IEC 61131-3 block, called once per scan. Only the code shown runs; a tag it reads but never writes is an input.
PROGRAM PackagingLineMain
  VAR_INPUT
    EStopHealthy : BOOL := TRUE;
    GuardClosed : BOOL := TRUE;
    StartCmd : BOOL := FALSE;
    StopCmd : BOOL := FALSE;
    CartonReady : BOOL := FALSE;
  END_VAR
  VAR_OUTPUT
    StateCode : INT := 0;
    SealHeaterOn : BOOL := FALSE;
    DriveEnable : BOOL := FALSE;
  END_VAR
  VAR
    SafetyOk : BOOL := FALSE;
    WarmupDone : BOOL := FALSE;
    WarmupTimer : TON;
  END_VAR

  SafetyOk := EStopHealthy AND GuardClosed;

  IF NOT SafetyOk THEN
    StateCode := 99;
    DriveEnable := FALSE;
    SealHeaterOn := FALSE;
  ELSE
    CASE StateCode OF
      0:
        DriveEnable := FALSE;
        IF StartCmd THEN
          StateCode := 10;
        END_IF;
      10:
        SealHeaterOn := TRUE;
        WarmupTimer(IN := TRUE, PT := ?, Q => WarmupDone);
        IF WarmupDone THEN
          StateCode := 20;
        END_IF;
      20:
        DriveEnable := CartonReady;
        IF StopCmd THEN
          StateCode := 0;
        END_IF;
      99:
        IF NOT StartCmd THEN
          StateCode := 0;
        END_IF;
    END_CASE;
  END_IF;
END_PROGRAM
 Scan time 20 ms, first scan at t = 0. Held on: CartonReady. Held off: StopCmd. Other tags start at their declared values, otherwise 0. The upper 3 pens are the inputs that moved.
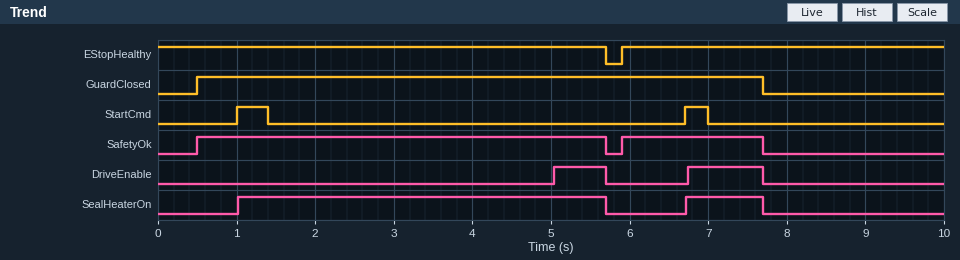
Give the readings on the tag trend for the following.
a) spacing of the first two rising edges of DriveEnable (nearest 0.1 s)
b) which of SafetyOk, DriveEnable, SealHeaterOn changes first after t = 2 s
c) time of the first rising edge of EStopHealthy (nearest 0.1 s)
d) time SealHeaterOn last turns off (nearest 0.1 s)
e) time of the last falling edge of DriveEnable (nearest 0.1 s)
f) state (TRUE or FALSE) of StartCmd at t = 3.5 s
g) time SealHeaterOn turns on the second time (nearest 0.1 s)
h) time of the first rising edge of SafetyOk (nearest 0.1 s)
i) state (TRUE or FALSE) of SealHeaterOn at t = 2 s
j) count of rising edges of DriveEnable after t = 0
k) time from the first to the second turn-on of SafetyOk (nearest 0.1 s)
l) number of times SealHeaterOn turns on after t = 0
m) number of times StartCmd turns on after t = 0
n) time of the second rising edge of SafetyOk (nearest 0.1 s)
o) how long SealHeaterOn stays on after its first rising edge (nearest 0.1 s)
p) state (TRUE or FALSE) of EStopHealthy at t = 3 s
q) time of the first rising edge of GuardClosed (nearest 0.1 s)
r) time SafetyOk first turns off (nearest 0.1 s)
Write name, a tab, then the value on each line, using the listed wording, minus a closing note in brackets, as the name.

spacing of the first two rising edges of DriveEnable	1.7 s
which of SafetyOk, DriveEnable, SealHeaterOn changes first after t = 2 s	DriveEnable
time of the first rising edge of EStopHealthy	5.9 s
time SealHeaterOn last turns off	7.7 s
time of the last falling edge of DriveEnable	7.7 s
state (TRUE or FALSE) of StartCmd at t = 3.5 s	FALSE
time SealHeaterOn turns on the second time	6.7 s
time of the first rising edge of SafetyOk	0.5 s
state (TRUE or FALSE) of SealHeaterOn at t = 2 s	TRUE
count of rising edges of DriveEnable after t = 0	2
time from the first to the second turn-on of SafetyOk	5.4 s
number of times SealHeaterOn turns on after t = 0	2
number of times StartCmd turns on after t = 0	2
time of the second rising edge of SafetyOk	5.9 s
how long SealHeaterOn stays on after its first rising edge	4.7 s
state (TRUE or FALSE) of EStopHealthy at t = 3 s	TRUE
time of the first rising edge of GuardClosed	0.5 s
time SafetyOk first turns off	5.7 s
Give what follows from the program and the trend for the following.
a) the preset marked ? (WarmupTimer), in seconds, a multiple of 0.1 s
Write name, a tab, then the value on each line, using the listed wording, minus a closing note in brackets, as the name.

the preset marked ? (WarmupTimer), in seconds, a multiple of 0.1 s	4.0 s
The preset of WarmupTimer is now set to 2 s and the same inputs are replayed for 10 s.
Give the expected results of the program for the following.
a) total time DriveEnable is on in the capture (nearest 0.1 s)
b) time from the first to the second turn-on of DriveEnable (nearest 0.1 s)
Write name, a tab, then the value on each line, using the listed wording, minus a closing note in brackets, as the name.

total time DriveEnable is on in the capture	3.6 s
time from the first to the second turn-on of DriveEnable	3.7 s
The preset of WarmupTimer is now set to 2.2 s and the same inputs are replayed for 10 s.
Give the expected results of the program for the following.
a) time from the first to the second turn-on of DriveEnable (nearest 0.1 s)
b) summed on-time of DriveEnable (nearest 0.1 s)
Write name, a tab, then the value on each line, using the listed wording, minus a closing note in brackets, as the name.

time from the first to the second turn-on of DriveEnable	3.5 s
summed on-time of DriveEnable	3.4 s
